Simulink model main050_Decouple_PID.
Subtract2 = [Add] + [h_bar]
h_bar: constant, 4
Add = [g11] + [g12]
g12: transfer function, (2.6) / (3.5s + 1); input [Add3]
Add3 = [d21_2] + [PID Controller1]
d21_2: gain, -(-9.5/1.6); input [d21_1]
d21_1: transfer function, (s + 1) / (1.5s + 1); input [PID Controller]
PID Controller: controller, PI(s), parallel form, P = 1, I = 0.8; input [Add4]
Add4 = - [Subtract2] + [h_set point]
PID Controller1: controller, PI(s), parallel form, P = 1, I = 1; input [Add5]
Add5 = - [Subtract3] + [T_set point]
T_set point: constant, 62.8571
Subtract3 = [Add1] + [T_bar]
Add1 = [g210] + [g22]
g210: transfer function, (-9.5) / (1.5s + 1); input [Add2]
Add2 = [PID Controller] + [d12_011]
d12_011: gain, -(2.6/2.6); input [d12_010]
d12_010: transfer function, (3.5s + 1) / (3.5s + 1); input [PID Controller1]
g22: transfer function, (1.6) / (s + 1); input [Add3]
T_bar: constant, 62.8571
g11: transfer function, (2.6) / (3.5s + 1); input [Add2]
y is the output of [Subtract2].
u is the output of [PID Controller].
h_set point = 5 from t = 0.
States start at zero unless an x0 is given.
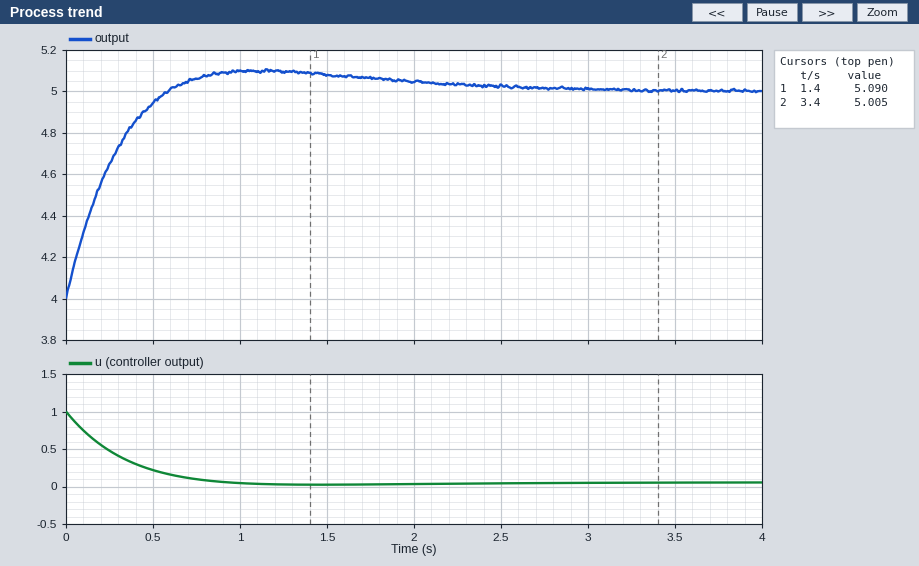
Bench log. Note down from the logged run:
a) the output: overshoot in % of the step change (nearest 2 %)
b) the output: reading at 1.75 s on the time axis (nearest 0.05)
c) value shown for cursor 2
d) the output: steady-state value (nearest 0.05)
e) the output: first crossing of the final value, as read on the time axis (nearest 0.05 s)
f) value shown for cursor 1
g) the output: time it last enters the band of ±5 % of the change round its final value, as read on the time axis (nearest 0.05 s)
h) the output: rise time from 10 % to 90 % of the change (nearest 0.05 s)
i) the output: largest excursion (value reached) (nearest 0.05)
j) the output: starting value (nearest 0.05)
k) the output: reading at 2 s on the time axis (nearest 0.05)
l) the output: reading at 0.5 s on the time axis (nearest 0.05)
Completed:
10 %
5.05
5.005
5.00
0.60 s
5.090
1.95 s
0.40 s
5.10
4.00
5.05
4.95
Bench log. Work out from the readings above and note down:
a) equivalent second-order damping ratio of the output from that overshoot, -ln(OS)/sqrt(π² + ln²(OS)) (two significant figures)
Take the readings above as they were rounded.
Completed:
0.59
